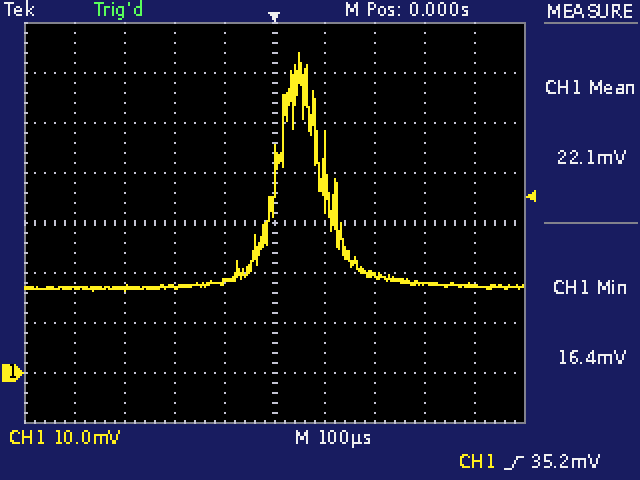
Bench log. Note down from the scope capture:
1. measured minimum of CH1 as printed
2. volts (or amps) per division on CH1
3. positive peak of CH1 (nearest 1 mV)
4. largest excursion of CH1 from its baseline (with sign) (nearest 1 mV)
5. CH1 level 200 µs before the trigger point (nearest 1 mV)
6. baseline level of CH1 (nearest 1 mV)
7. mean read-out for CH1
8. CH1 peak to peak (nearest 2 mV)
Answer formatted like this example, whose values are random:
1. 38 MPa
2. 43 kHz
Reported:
1. 16.4 mV
2. 10 mV
3. 64 mV
4. +47 mV
5. 17 mV
6. 17 mV
7. 22.1 mV
8. 48 mV
